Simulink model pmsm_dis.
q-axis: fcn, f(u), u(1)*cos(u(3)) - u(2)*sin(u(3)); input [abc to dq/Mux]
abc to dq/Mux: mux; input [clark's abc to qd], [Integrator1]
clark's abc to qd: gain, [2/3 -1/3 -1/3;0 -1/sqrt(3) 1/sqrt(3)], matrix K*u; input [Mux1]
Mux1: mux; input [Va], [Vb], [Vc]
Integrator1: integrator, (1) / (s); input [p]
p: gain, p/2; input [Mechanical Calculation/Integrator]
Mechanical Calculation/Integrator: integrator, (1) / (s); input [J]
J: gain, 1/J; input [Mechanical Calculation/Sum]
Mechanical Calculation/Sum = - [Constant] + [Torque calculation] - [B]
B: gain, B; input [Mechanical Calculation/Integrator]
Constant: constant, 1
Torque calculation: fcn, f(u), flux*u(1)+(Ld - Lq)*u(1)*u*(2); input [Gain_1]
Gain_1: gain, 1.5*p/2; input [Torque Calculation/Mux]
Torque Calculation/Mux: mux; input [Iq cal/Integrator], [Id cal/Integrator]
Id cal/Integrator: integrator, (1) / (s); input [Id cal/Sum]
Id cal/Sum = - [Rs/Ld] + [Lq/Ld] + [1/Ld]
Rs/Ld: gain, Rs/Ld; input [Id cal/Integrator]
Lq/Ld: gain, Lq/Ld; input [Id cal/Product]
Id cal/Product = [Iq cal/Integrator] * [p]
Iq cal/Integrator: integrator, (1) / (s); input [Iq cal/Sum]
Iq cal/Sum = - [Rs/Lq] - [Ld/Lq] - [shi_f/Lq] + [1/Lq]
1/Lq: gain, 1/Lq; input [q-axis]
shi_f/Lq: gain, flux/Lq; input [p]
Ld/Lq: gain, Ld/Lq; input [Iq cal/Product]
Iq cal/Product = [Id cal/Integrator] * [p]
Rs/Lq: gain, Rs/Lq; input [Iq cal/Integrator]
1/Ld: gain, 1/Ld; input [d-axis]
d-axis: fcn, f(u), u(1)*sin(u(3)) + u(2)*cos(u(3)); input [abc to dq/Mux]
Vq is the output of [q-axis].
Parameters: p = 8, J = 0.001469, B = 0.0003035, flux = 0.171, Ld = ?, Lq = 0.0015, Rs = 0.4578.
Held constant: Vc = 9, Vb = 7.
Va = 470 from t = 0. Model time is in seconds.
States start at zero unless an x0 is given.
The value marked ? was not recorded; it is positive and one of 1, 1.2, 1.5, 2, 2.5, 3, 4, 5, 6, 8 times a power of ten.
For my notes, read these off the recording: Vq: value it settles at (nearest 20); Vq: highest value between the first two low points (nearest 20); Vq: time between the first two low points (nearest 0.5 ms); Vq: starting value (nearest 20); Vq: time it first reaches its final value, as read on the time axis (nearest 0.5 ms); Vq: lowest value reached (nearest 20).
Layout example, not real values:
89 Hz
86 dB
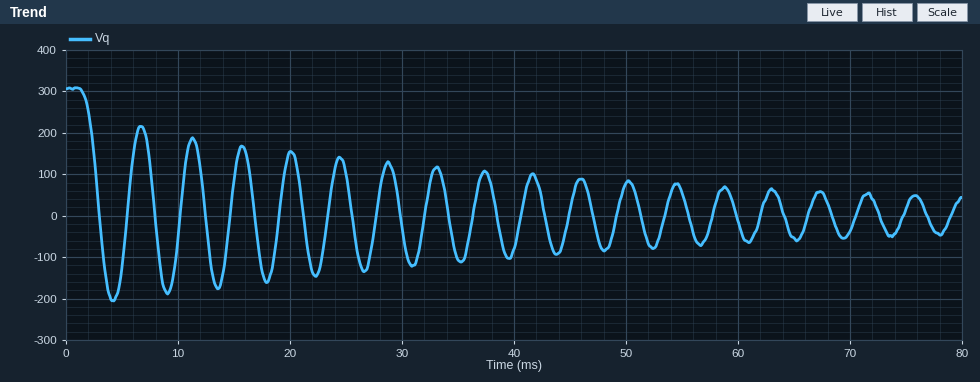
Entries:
0
220
5.0 ms
300
3.0 ms
-200
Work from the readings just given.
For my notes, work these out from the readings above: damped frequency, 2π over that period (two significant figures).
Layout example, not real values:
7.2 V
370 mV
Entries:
1.3 rad/ms
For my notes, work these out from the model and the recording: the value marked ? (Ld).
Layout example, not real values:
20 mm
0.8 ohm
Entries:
0.0015
